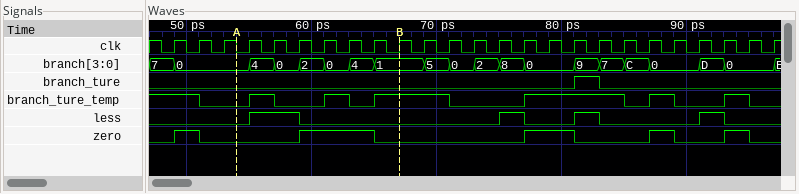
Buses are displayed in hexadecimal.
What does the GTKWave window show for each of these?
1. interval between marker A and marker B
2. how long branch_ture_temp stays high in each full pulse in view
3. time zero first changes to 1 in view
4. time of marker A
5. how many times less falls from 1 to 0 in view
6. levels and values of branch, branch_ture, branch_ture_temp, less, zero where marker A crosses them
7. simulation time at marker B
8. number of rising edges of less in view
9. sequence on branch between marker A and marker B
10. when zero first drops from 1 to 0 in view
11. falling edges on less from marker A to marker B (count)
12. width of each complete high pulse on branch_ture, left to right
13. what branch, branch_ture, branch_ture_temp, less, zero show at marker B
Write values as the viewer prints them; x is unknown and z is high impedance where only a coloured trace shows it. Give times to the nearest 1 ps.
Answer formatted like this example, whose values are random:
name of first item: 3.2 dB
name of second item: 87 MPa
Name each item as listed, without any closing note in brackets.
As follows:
interval between marker A and marker B: 13 ps
how long branch_ture_temp stays high in each full pulse in view: 2 ps, 2 ps, 6 ps, 8 ps, 2 ps, 2 ps
time zero first changes to 1 in view: 49 ps
time of marker A: 54 ps
how many times less falls from 1 to 0 in view: 4
levels and values of branch, branch_ture, branch_ture_temp, less, zero where marker A crosses them: branch=0, branch_ture=0, branch_ture_temp=0, less=0, zero=0
simulation time at marker B: 67 ps
number of rising edges of less in view: 4
sequence on branch between marker A and marker B: 0, 4, 0, 2, 0, 4, 1
when zero first drops from 1 to 0 in view: 51 ps
falling edges on less from marker A to marker B: 1
width of each complete high pulse on branch_ture, left to right: 2 ps
what branch, branch_ture, branch_ture_temp, less, zero show at marker B: branch=1, branch_ture=0, branch_ture_temp=1, less=0, zero=0
